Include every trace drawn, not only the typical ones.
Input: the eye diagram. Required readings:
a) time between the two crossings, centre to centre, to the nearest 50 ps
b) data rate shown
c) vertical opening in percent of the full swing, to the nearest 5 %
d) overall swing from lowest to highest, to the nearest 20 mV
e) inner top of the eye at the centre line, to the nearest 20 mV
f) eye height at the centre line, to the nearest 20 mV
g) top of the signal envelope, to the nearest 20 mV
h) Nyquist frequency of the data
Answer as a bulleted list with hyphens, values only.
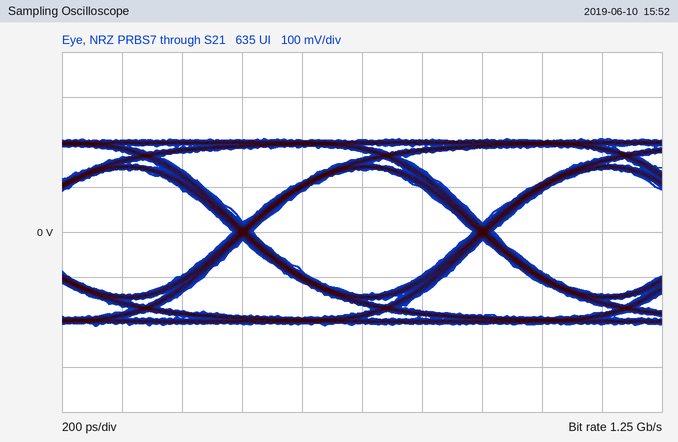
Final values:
- 800 ps
- 1.25 Gb/s
- 65 %
- 420 mV
- 140 mV
- 280 mV
- 200 mV
- 625 MHz
